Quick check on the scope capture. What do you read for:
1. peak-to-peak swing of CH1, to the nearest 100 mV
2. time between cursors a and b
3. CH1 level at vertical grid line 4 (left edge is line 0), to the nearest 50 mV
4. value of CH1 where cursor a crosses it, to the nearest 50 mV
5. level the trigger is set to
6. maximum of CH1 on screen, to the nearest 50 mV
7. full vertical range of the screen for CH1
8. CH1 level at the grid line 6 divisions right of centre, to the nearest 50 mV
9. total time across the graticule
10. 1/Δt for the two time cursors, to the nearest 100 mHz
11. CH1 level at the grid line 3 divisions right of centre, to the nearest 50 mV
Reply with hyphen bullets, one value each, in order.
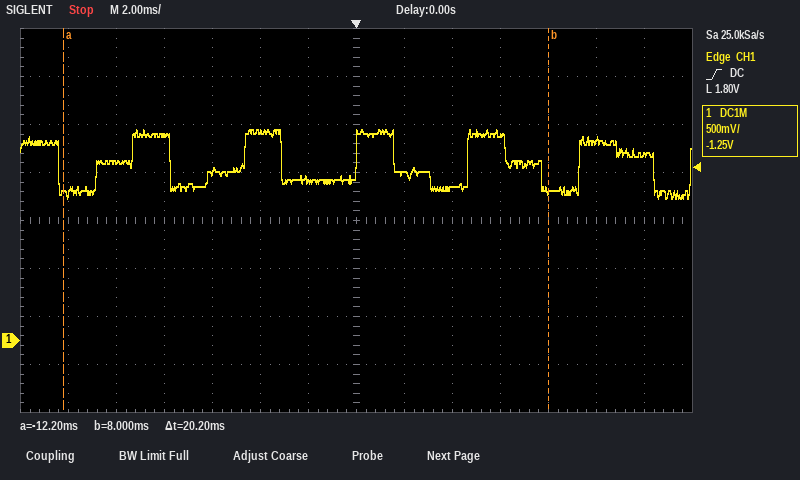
- 700 mV
- 20.2 ms
- 1.75 V
- 1.55 V
- 1.80 V
- 2.20 V
- 4 V
- 1.95 V
- 28 ms
- 49.5 Hz
- 2.15 V
